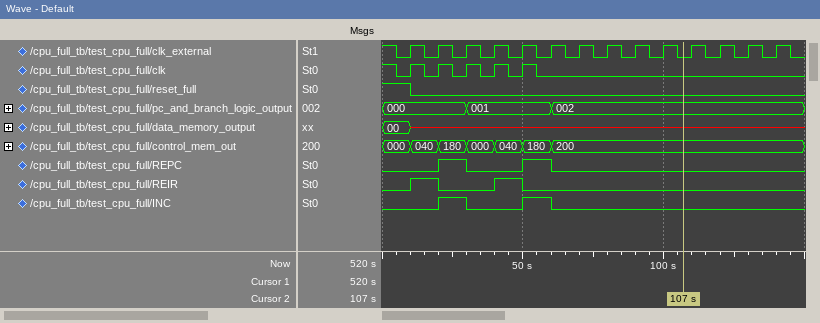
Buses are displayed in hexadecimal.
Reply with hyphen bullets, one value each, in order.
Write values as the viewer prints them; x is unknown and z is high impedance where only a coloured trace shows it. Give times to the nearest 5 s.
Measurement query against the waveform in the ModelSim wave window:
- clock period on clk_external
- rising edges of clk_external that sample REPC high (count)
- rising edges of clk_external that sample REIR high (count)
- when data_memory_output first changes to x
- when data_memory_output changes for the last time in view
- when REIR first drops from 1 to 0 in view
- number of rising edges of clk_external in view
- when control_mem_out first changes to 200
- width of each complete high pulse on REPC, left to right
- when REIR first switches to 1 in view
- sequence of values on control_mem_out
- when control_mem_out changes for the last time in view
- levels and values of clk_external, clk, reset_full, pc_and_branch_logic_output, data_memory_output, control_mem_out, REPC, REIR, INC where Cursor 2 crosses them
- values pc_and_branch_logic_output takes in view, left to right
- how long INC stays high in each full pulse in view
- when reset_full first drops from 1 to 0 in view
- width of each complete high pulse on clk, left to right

- 10 s
- 2
- 2
- 10 s
- 10 s
- 20 s
- 14
- 60 s
- 10 s, 10 s
- 10 s
- 000, 040, 180, 000, 040, 180, 200
- 60 s
- clk_external=0, clk=0, reset_full=0, pc_and_branch_logic_output=002, data_memory_output=x, control_mem_out=200, REPC=0, REIR=0, INC=0
- 000, 001, 002
- 10 s, 10 s
- 10 s
- 5 s, 5 s, 5 s, 5 s, 5 s
